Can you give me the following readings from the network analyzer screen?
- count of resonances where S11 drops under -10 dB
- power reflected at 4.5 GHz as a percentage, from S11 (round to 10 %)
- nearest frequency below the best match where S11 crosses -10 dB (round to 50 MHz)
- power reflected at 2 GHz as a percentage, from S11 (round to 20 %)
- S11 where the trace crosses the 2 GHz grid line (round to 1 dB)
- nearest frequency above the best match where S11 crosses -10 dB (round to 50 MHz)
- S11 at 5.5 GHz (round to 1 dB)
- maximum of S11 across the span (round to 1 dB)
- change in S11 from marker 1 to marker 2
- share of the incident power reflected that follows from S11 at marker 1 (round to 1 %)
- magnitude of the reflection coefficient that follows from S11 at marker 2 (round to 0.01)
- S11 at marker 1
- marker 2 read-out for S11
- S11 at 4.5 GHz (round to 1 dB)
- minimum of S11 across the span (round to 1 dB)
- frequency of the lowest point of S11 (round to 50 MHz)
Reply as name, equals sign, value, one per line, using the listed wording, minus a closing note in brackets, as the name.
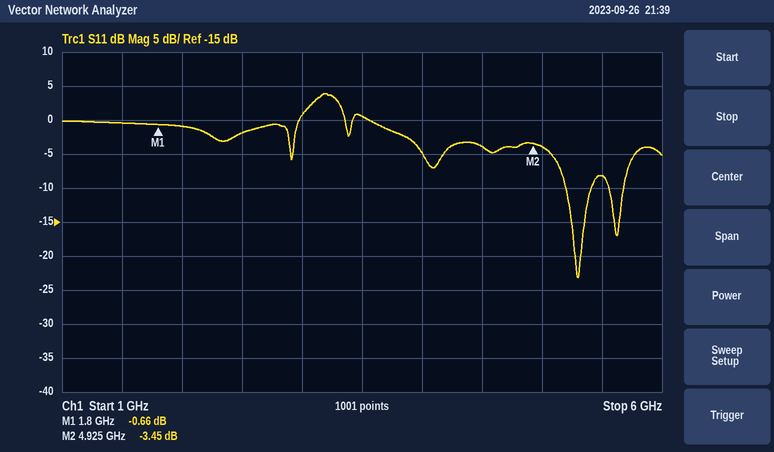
count of resonances where S11 drops under -10 dB = 2
power reflected at 4.5 GHz as a percentage, from S11 = 40 %
nearest frequency below the best match where S11 crosses -10 dB = 5.20 GHz
power reflected at 2 GHz as a percentage, from S11 = 80 %
S11 where the trace crosses the 2 GHz grid line = -1 dB
nearest frequency above the best match where S11 crosses -10 dB = 5.40 GHz
S11 at 5.5 GHz = -8 dB
maximum of S11 across the span = 4 dB
change in S11 from marker 1 to marker 2 = -2.79 dB
share of the incident power reflected that follows from S11 at marker 1 = 86 %
magnitude of the reflection coefficient that follows from S11 at marker 2 = 0.67
S11 at marker 1 = -0.66 dB
marker 2 read-out for S11 = -3.45 dB
S11 at 4.5 GHz = -4 dB
minimum of S11 across the span = -23 dB
frequency of the lowest point of S11 = 5.30 GHz
